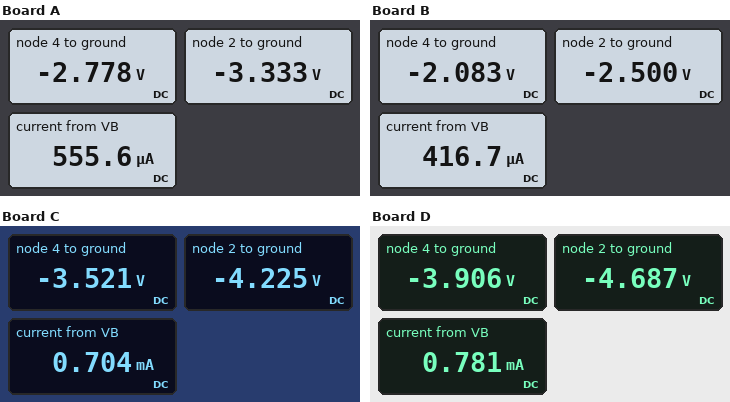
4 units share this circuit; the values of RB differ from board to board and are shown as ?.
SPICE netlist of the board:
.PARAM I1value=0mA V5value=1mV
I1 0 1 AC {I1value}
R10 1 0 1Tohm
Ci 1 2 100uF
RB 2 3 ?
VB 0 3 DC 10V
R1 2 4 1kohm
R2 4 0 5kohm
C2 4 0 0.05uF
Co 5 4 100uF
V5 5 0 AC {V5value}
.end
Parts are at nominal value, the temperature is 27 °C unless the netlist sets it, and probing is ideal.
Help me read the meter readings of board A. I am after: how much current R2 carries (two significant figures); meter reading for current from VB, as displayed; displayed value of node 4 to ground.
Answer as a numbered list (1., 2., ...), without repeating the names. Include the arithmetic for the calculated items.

1. (0 V - (-2.778 V)) / 5 kΩ = 560 µA
2. 555.6 µA
3. -2.778 V
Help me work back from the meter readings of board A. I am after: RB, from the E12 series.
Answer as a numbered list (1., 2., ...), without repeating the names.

1. 12 kΩ
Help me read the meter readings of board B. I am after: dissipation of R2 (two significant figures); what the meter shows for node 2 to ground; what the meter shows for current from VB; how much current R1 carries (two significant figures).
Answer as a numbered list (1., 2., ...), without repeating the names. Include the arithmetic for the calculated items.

1. (0 V - (-2.083 V))^2 / 5 kΩ = 870 µW
2. -2.500 V
3. 416.7 µA
4. (-2.083 V - (-2.5 V)) / 1 kΩ = 420 µA
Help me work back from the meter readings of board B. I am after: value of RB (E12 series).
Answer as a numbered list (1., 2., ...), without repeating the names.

1. 18 kΩ
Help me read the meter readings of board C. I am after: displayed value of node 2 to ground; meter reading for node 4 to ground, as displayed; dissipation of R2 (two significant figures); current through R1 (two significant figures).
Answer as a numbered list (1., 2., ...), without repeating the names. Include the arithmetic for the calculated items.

1. -4.225 V
2. -3.521 V
3. (0 V - (-3.521 V))^2 / 5 kΩ = 2.5 mW
4. (-3.521 V - (-4.225 V)) / 1 kΩ = 700 µA
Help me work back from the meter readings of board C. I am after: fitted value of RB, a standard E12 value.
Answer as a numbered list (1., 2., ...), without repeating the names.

1. 8.2 kΩ
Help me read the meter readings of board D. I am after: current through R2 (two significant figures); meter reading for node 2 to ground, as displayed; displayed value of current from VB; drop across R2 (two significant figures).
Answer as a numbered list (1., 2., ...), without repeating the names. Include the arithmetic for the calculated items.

1. (0 V - (-3.906 V)) / 5 kΩ = 780 µA
2. -4.687 V
3. 0.781 mA
4. 0 V - (-3.906 V) = 3.9 V
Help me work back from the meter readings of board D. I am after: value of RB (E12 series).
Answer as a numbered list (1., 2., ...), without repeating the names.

1. 6.8 kΩ
